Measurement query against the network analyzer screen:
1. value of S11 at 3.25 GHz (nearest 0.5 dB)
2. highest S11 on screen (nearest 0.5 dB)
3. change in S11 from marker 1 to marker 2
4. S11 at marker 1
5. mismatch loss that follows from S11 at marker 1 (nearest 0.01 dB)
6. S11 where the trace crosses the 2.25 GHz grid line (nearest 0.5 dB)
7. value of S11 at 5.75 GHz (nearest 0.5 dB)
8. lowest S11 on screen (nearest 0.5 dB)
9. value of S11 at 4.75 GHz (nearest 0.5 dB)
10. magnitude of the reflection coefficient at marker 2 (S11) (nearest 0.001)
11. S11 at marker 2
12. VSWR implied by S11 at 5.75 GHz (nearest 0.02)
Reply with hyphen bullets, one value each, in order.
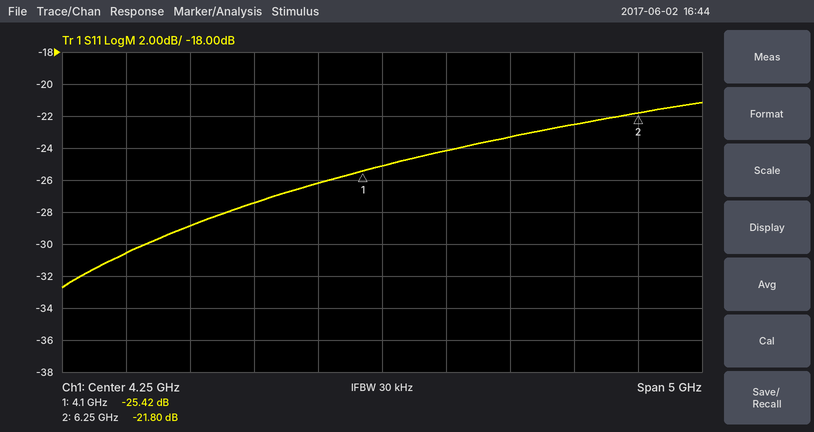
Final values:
- -27.5 dB
- -21.0 dB
- 3.62 dB
- -25.42 dB
- 0.01 dB
- -30.5 dB
- -22.5 dB
- -32.5 dB
- -24.0 dB
- 0.081
- -21.80 dB
- 1.16
